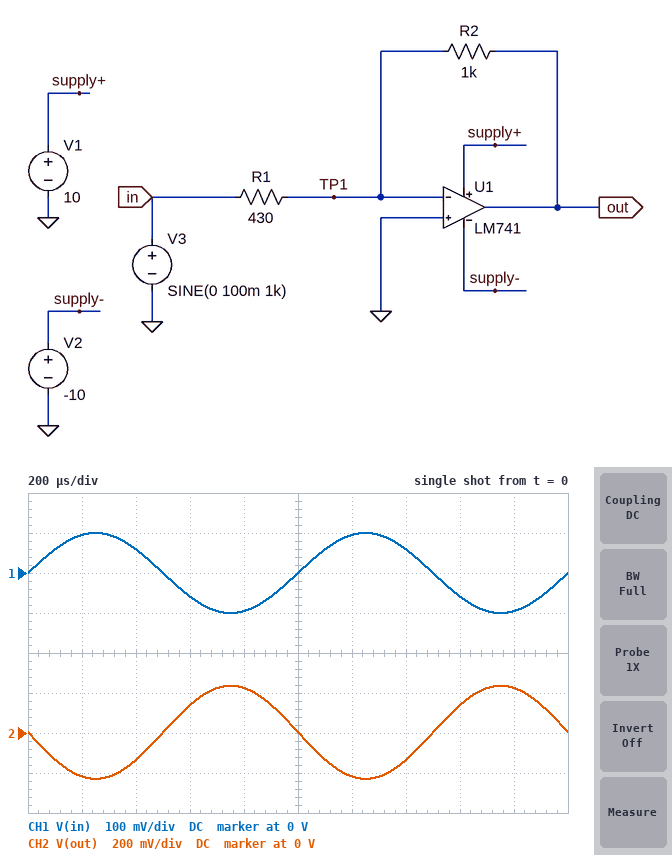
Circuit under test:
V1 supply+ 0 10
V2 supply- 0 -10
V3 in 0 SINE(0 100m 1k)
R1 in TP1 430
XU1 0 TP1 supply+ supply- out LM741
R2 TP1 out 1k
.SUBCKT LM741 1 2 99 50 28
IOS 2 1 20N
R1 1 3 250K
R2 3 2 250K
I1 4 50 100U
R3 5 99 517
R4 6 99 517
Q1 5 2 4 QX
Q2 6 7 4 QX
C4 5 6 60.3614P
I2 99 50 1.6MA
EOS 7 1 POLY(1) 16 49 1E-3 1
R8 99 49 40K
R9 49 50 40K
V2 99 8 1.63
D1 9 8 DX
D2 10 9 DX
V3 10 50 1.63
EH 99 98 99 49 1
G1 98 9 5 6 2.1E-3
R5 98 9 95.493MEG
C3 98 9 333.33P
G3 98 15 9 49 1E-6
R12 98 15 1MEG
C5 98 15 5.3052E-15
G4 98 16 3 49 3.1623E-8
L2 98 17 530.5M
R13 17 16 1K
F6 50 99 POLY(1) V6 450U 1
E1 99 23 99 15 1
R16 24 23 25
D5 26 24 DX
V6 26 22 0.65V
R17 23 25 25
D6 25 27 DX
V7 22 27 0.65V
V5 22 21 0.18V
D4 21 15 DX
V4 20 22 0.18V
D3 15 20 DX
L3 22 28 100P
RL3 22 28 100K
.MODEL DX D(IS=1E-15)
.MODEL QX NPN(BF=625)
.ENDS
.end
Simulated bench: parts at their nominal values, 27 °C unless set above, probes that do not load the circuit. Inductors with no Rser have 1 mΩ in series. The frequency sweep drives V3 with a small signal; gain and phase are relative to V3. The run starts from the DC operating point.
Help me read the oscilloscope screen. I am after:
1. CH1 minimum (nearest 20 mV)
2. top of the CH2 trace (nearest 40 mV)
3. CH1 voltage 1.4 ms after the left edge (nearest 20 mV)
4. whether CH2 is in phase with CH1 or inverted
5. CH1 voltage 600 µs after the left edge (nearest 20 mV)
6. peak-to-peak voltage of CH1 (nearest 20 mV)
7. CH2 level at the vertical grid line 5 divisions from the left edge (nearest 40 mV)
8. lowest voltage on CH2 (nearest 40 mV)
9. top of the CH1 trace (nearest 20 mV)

-100 mV
240 mV
60 mV
inverted
-60 mV
200 mV
0 V
-240 mV
100 mV
